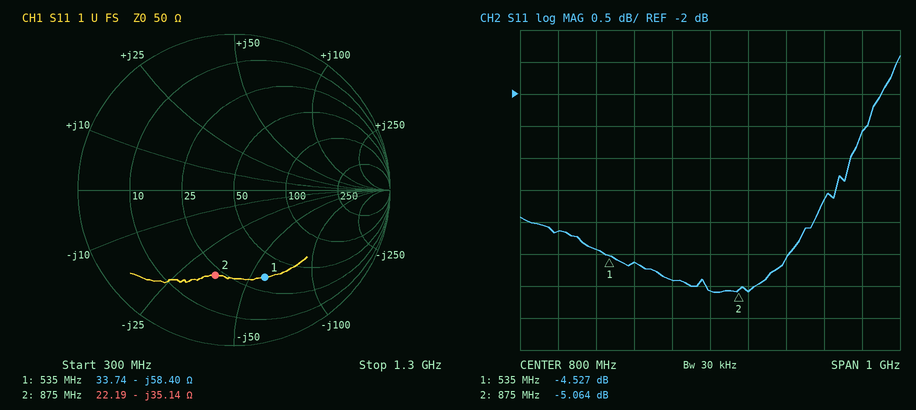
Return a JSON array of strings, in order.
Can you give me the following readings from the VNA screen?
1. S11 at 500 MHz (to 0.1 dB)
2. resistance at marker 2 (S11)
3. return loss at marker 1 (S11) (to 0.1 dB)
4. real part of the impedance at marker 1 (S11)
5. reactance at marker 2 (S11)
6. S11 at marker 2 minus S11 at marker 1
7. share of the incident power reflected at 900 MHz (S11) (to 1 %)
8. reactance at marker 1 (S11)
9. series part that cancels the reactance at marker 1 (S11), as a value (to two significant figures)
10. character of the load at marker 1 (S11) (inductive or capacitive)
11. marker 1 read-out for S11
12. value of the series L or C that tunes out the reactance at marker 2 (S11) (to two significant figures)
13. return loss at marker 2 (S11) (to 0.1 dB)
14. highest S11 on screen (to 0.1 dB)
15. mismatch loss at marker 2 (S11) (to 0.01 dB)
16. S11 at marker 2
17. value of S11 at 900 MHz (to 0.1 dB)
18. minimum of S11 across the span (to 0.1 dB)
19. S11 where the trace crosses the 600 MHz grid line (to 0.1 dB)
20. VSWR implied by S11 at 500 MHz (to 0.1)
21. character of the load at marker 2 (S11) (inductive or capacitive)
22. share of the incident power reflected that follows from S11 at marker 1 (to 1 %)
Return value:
["-4.4 dB", "22.19 Ω", "4.5 dB", "33.74 Ω", "-35.14 Ω", "-0.537 dB", "31 %", "-58.40 Ω", "17 nH", "capacitive", "-4.527 dB", "6.4 nH", "5.1 dB", "-1.4 dB", "1.62 dB", "-5.064 dB", "-5.1 dB", "-5.1 dB", "-4.6 dB", "4.0", "capacitive", "35 %"]
